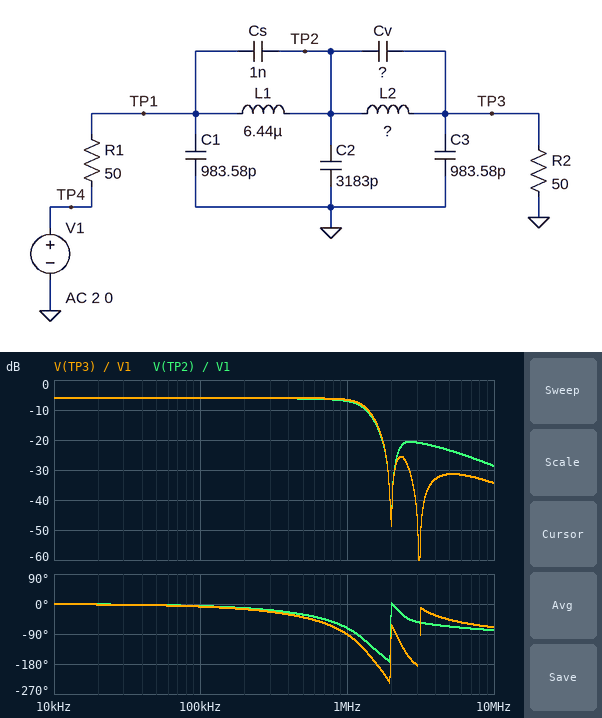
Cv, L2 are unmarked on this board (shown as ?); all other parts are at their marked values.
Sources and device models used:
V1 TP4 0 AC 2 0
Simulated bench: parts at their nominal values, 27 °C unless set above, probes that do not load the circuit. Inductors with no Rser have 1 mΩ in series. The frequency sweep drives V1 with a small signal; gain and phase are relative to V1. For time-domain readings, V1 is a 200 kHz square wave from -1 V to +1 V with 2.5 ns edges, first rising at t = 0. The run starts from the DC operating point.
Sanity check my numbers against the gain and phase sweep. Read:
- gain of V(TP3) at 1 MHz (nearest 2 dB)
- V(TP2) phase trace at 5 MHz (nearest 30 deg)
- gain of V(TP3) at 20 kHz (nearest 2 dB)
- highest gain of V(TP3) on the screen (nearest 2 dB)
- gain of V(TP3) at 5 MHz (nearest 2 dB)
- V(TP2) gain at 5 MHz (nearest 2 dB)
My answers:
-6 dB
-60 deg
-6 dB
-6 dB
-32 dB
-24 dB
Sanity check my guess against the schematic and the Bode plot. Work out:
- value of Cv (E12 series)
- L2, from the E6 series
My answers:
1.2 nF
2.2 µH
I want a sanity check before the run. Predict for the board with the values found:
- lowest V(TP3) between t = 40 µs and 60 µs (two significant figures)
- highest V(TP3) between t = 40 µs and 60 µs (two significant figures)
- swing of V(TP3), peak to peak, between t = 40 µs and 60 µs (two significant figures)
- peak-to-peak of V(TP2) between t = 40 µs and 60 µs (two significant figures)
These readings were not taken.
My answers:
-630 mV
630 mV
1.3 V
1.2 V
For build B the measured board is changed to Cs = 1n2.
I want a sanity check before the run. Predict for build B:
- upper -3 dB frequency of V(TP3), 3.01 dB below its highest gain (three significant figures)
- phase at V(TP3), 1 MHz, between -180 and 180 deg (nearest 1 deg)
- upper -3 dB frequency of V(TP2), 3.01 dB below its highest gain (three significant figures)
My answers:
1.25 MHz
-94 deg
1.21 MHz
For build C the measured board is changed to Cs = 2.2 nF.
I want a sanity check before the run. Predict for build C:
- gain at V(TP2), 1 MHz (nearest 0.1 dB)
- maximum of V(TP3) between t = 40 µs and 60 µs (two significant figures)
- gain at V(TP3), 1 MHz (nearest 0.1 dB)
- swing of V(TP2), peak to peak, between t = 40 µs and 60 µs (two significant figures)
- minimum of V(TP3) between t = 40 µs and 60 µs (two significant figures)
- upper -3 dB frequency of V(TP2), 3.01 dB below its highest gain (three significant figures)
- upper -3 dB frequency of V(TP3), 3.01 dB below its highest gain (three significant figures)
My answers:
-8.8 dB
680 mV
-8.4 dB
1.3 V
-680 mV
1.01 MHz
1.03 MHz
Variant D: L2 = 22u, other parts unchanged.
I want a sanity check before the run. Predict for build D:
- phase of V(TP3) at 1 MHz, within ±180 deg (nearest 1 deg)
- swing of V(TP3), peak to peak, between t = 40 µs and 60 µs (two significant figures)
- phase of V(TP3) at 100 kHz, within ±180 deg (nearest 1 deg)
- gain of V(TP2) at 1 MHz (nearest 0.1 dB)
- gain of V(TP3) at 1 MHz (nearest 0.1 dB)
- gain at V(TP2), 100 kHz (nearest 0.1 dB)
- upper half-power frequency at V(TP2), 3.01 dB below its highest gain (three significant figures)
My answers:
-24 deg
1.2 V
-15 deg
0.1 dB
-36.7 dB
-5.8 dB
1.17 MHz
